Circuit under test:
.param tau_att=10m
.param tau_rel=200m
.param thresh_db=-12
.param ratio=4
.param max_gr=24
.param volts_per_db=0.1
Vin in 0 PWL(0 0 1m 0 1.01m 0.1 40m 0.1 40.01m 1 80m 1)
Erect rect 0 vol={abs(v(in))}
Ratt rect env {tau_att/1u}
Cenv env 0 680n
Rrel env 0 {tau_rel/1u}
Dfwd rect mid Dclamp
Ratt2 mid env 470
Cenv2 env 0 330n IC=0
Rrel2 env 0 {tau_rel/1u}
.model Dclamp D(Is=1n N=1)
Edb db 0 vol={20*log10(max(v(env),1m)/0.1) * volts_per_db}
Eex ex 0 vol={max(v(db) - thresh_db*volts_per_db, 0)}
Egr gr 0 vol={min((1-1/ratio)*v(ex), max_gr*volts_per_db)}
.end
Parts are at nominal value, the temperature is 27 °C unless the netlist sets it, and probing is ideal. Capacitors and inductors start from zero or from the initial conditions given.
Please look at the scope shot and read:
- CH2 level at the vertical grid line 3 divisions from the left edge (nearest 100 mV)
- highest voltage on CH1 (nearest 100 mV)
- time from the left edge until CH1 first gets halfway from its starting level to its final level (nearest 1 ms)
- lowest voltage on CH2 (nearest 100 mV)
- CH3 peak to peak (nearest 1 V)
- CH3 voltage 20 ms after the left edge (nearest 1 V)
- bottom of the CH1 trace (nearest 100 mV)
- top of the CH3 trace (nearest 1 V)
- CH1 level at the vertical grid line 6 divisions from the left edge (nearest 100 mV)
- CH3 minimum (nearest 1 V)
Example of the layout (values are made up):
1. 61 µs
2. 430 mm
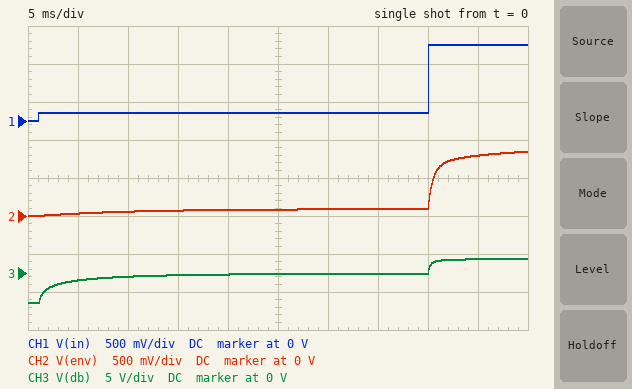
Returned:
1. 100 mV
2. 1.0 V
3. 40 ms
4. 0 V
5. 6 V
6. 0 V
7. 0 V
8. 2 V
9. 100 mV
10. -4 V
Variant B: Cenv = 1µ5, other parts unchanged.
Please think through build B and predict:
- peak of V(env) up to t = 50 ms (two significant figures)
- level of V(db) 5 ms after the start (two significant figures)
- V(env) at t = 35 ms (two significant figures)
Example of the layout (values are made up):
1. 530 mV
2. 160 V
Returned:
1. 800 mV
2. -1.4 V
3. 79 mV
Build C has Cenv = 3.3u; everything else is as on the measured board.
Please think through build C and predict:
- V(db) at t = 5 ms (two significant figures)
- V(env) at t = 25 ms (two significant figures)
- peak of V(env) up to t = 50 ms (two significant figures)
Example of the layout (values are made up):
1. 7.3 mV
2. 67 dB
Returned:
1. -2.0 V
2. 47 mV
3. 750 mV
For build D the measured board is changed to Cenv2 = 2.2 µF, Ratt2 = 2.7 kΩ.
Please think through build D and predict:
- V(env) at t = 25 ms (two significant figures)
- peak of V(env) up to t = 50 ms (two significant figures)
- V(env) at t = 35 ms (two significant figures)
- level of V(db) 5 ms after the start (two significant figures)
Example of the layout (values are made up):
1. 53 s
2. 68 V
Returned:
1. 55 mV
2. 630 mV
3. 66 mV
4. -1.8 V
